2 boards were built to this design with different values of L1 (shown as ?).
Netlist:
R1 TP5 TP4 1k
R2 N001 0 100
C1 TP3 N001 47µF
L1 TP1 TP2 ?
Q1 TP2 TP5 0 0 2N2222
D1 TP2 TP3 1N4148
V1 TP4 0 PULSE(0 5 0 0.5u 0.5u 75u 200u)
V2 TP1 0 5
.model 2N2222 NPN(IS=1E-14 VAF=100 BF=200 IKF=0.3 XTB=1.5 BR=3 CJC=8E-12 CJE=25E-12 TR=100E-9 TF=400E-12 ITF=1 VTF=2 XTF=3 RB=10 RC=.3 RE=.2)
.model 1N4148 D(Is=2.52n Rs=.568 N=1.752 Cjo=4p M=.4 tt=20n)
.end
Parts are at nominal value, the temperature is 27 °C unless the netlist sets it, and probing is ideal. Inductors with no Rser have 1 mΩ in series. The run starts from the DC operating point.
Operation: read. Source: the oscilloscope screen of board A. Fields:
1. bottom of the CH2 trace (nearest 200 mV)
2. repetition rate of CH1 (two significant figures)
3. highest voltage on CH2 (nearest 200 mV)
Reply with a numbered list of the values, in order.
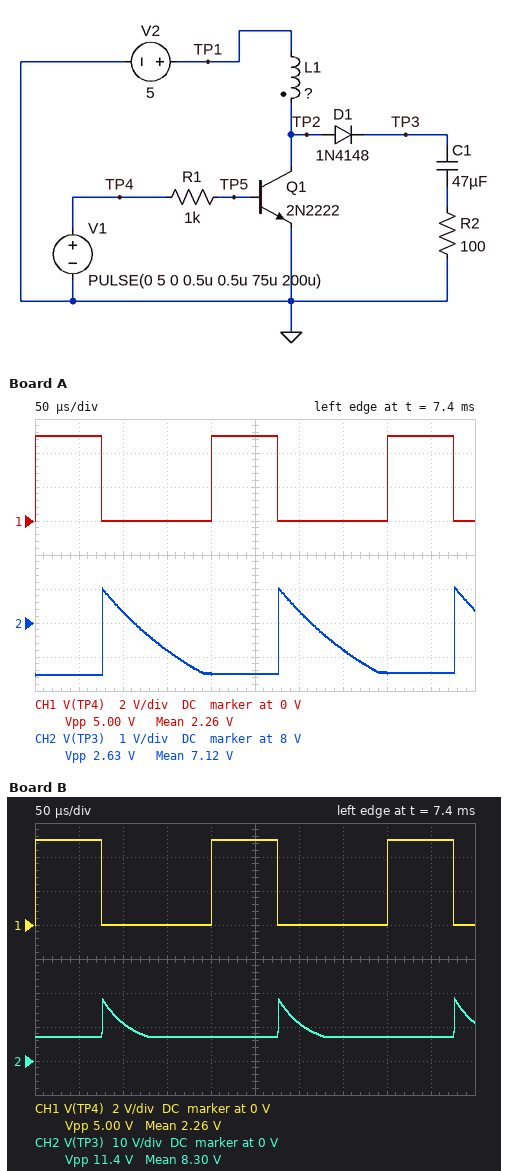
1. 6.4 V
2. 5.0 kHz
3. 9.0 V
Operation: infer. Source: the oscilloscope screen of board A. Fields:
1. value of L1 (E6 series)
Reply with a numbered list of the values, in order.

1. 15 mH
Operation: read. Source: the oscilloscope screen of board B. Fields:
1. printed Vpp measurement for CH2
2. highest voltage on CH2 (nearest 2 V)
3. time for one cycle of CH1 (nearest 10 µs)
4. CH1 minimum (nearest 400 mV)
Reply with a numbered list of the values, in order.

1. 11.4 V
2. 18 V
3. 200 µs
4. 0 V
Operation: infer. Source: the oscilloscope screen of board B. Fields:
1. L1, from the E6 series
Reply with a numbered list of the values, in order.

1. 3.3 mH
